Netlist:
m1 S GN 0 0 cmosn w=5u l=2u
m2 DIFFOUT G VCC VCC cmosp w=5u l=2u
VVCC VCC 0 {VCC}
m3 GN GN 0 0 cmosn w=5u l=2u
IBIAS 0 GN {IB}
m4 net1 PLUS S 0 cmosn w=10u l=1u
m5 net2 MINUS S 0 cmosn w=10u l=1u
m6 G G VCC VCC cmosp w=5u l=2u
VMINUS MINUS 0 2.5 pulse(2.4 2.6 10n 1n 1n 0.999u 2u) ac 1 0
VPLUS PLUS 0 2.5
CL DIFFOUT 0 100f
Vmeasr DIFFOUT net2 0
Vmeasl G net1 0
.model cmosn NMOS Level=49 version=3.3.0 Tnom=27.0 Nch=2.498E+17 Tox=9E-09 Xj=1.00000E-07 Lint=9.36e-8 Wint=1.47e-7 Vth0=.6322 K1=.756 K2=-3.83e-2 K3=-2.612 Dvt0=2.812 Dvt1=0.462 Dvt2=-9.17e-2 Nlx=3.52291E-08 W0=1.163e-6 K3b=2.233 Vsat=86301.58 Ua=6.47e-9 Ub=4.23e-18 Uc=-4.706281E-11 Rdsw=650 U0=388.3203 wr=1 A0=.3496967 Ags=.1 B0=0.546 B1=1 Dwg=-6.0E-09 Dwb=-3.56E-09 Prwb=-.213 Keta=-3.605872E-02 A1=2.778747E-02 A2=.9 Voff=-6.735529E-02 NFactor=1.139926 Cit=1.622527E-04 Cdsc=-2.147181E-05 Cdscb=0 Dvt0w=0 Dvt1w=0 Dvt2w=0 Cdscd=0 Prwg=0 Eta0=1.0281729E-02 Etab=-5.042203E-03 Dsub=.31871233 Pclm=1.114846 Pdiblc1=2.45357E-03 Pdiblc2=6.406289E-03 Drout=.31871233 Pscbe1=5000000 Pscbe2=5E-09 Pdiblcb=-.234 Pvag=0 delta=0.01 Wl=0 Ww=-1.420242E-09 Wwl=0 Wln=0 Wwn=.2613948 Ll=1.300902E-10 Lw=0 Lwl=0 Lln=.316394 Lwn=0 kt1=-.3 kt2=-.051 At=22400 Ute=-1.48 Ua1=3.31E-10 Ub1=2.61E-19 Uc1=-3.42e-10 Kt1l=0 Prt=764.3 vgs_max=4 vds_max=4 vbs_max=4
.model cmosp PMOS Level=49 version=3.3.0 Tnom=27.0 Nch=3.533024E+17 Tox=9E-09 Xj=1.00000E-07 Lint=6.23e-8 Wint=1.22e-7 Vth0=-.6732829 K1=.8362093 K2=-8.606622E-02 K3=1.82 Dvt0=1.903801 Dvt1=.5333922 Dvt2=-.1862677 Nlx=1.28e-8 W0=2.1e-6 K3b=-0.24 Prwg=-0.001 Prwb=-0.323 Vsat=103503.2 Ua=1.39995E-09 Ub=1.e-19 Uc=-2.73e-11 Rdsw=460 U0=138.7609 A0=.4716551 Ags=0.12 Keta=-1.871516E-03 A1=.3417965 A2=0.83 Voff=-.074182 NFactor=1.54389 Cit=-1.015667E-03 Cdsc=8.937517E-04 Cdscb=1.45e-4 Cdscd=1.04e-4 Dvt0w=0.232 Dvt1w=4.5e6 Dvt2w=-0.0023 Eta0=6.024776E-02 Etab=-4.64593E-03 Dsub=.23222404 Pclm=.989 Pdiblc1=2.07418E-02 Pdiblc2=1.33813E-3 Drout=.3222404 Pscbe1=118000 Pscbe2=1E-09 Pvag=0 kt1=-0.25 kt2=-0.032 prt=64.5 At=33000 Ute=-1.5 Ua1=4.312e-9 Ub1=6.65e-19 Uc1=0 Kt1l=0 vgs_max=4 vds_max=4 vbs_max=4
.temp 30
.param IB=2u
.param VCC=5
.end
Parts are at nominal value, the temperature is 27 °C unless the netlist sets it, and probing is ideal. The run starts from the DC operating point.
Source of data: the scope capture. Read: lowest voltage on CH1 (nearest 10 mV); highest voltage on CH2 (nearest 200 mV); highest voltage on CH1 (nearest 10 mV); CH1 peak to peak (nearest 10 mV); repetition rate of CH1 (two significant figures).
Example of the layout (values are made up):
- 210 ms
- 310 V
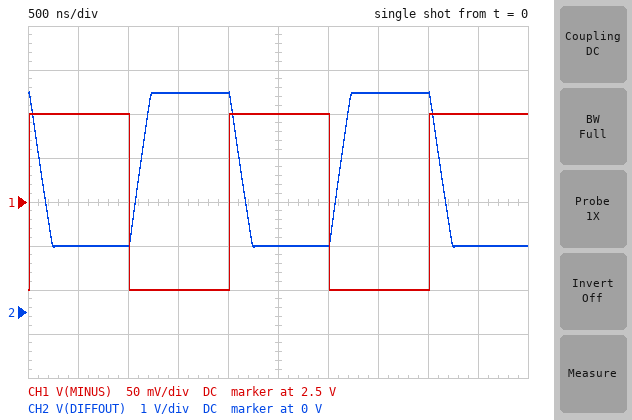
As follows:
- 2.40 V
- 5.0 V
- 2.60 V
- 200 mV
- 500 kHz
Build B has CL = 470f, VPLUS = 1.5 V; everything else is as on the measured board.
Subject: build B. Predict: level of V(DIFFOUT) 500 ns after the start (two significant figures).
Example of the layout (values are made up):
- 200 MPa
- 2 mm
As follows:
- 660 mV
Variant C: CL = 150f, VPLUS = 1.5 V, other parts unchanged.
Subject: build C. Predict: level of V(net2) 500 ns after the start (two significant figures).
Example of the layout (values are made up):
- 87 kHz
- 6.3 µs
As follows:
- 660 mV
